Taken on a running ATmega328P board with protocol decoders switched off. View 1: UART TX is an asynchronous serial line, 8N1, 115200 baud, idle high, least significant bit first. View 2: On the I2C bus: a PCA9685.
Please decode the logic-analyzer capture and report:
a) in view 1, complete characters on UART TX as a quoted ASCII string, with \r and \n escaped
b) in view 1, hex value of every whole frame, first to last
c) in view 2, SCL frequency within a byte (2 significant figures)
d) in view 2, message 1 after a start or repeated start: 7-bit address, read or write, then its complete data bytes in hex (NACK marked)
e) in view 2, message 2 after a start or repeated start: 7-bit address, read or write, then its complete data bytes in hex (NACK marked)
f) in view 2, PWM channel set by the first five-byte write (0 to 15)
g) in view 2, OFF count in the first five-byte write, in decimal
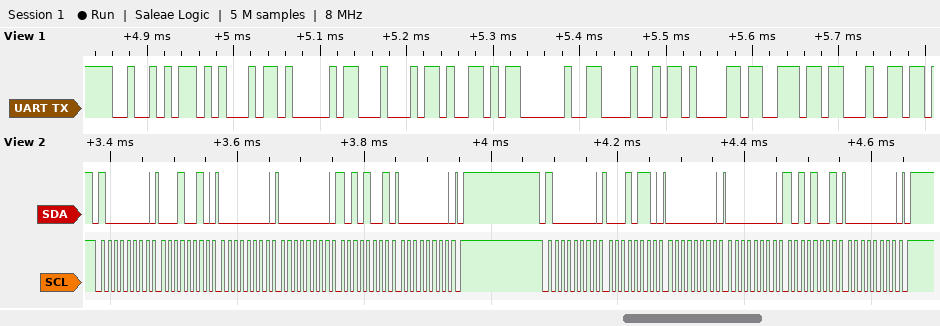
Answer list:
"READY Hand"
52 45 41 44 59 20 48 61 6E 64
100 kHz
0x40 write: 12 00 00 A9 00
0x40 write: 16 00 00 A9 00
3
169
